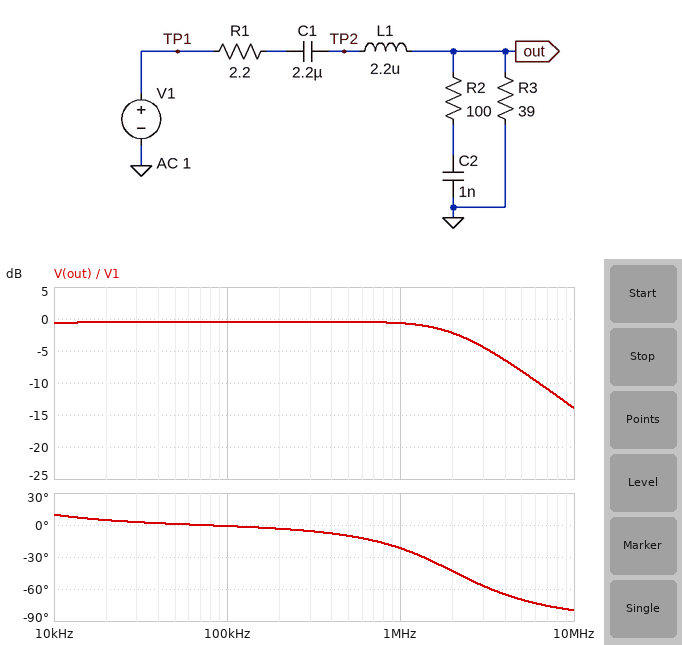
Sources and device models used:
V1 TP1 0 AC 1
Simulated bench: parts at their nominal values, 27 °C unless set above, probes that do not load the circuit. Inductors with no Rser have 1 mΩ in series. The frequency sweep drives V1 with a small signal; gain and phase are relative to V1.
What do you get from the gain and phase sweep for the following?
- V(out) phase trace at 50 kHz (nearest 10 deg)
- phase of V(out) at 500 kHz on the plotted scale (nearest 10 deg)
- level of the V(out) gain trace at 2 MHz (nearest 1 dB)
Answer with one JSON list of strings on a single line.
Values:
["0 deg", "-10 deg", "-2 dB"]
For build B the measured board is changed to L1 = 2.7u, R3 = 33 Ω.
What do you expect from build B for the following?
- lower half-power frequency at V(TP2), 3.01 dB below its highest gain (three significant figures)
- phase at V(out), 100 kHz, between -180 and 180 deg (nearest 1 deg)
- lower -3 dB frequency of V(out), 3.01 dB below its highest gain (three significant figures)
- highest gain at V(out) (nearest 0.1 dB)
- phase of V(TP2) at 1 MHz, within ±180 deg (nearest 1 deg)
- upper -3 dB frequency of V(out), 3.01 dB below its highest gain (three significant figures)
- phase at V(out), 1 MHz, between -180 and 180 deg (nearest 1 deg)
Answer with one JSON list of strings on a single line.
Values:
["2.36 kHz", "-2 deg", "2.05 kHz", "-0.6 dB", "2 deg", "1.93 MHz", "-30 deg"]
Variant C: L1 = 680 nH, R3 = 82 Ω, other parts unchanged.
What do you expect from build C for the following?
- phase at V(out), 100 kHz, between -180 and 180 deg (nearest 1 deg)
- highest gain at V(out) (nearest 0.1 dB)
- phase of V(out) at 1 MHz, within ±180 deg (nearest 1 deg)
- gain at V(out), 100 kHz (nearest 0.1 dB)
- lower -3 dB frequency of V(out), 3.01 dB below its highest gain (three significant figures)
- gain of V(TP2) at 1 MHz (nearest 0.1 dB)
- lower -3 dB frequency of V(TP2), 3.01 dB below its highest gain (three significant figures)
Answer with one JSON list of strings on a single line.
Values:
["0 deg", "-0.1 dB", "-4 deg", "-0.2 dB", "885 Hz", "-0.3 dB", "908 Hz"]
